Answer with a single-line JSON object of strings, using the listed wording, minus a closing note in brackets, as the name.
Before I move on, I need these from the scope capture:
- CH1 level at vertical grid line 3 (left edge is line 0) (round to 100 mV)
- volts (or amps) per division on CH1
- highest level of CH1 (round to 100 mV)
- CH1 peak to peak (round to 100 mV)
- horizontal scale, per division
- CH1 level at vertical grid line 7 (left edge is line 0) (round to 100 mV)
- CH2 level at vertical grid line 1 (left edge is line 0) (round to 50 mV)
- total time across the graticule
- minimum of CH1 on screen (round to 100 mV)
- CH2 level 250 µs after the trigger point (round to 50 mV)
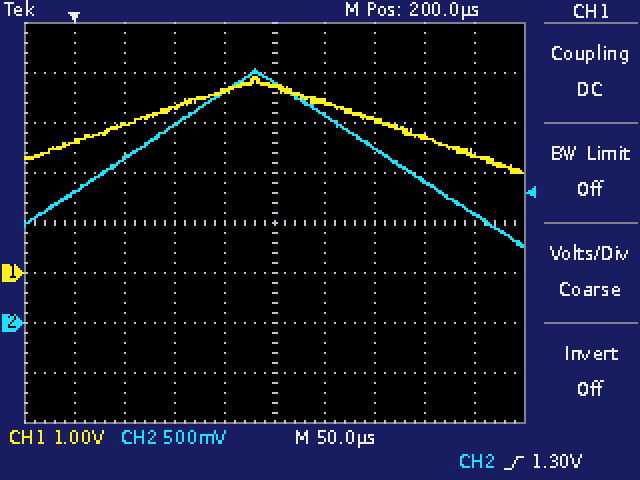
{"CH1 level at vertical grid line 3 (left edge is line 0)": "3.3 V", "volts (or amps) per division on CH1": "1 V", "highest level of CH1": "3.9 V", "CH1 peak to peak": "1.9 V", "horizontal scale, per division": "50 µs", "CH1 level at vertical grid line 7 (left edge is line 0)": "3.1 V", "CH2 level at vertical grid line 1 (left edge is line 0)": "1.30 V", "total time across the graticule": "500 µs", "minimum of CH1 on screen": "2.0 V", "CH2 level 250 µs after the trigger point": "2.10 V"}
